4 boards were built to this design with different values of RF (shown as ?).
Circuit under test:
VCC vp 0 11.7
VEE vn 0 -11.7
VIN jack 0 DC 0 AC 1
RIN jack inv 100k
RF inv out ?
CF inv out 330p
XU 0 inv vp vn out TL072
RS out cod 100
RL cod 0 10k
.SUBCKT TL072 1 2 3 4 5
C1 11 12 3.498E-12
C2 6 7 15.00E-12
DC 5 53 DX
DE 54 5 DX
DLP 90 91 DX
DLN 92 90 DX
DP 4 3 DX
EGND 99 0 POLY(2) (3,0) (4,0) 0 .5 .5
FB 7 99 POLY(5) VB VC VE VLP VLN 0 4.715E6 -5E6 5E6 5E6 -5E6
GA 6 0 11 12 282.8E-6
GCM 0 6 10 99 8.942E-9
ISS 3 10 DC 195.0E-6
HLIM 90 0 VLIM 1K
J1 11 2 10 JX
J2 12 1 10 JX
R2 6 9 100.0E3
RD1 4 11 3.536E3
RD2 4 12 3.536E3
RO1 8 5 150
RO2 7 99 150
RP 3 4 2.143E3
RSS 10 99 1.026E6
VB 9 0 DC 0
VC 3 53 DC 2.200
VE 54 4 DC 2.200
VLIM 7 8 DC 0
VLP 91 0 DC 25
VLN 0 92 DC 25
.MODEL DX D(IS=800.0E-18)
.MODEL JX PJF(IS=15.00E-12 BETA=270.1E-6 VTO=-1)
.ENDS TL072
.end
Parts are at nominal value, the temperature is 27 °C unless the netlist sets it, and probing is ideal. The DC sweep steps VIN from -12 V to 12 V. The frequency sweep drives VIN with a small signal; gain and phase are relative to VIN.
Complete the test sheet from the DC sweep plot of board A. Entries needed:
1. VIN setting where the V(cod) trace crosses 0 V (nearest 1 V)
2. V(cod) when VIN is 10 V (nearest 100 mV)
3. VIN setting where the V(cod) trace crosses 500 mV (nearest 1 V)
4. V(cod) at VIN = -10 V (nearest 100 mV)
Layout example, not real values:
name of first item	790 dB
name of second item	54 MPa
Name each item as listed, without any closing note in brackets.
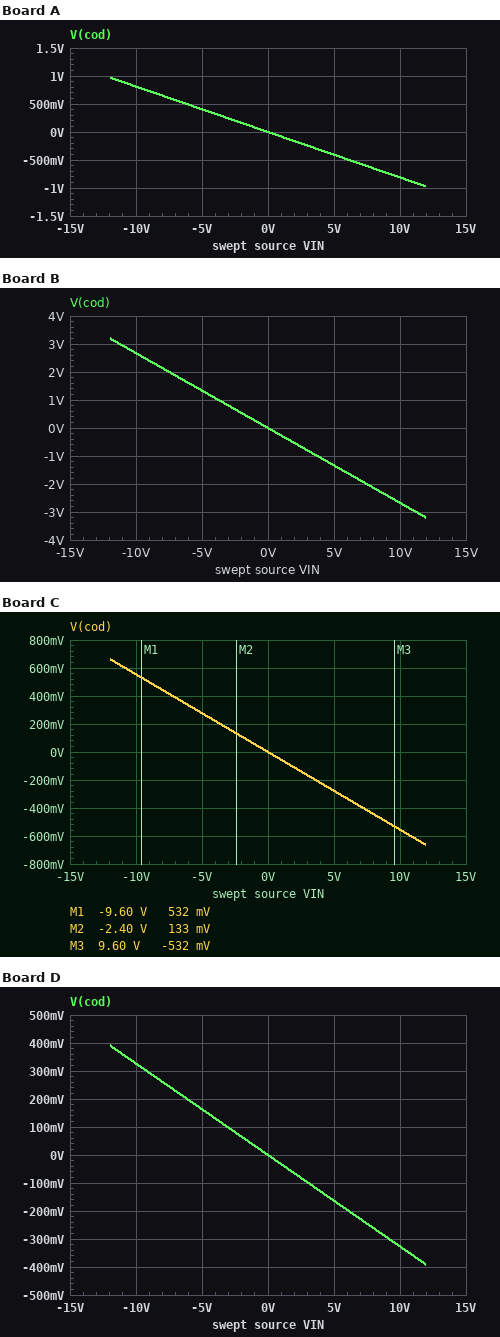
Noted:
VIN setting where the V(cod) trace crosses 0 V	0 V
V(cod) when VIN is 10 V	-800 mV
VIN setting where the V(cod) trace crosses 500 mV	-6 V
V(cod) at VIN = -10 V	800 mV
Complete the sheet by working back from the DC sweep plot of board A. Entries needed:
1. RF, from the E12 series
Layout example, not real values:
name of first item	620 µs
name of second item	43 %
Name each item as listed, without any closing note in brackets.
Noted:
RF, from the E12 series	8.2 kΩ
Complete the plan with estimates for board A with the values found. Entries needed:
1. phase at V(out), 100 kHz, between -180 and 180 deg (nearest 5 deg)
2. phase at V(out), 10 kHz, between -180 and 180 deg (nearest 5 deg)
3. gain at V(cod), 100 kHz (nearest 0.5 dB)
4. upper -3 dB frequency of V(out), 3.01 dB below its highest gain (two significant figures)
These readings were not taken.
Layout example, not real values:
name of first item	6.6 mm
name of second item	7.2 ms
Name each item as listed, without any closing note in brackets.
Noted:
phase at V(out), 100 kHz, between -180 and 180 deg	120 deg
phase at V(out), 10 kHz, between -180 and 180 deg	170 deg
gain at V(cod), 100 kHz	-27.5 dB
upper -3 dB frequency of V(out), 3.01 dB below its highest gain	59 kHz
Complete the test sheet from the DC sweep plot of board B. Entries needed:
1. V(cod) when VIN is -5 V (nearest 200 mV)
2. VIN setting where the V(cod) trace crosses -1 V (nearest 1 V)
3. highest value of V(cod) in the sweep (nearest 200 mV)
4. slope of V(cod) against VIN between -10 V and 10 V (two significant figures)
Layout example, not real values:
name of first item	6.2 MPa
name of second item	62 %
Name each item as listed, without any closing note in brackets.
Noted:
V(cod) when VIN is -5 V	1.4 V
VIN setting where the V(cod) trace crosses -1 V	4 V
highest value of V(cod) in the sweep	3.2 V
slope of V(cod) against VIN between -10 V and 10 V	-0.27 V/V
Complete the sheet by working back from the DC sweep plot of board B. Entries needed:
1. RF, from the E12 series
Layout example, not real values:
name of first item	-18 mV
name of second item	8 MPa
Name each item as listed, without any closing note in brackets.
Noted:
RF, from the E12 series	27 kΩ
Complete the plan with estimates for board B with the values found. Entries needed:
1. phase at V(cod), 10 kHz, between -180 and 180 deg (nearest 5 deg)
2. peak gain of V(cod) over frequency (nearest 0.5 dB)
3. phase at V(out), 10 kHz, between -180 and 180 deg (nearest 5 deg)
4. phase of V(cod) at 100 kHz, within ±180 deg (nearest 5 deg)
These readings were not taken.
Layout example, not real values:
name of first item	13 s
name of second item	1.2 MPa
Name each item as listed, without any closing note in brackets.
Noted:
phase at V(cod), 10 kHz, between -180 and 180 deg	150 deg
peak gain of V(cod) over frequency	-11.5 dB
phase at V(out), 10 kHz, between -180 and 180 deg	150 deg
phase of V(cod) at 100 kHz, within ±180 deg	100 deg
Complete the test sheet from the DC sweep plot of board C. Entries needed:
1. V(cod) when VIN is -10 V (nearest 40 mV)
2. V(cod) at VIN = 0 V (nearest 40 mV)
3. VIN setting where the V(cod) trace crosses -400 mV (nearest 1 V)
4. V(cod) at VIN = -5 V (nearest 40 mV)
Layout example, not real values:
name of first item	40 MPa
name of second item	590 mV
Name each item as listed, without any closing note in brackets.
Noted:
V(cod) when VIN is -10 V	560 mV
V(cod) at VIN = 0 V	0 V
VIN setting where the V(cod) trace crosses -400 mV	7 V
V(cod) at VIN = -5 V	280 mV
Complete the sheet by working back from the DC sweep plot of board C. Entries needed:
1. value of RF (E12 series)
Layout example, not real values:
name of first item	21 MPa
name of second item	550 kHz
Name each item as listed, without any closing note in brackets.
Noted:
value of RF	5.6 kΩ
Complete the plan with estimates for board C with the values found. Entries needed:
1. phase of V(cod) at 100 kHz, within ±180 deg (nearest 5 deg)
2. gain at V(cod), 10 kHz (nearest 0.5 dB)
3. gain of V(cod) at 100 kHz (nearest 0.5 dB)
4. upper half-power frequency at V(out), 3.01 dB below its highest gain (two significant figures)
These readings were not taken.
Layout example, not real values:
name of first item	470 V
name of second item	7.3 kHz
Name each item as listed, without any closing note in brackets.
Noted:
phase of V(cod) at 100 kHz, within ±180 deg	130 deg
gain at V(cod), 10 kHz	-25.0 dB
gain of V(cod) at 100 kHz	-29.0 dB
upper half-power frequency at V(out), 3.01 dB below its highest gain	86 kHz
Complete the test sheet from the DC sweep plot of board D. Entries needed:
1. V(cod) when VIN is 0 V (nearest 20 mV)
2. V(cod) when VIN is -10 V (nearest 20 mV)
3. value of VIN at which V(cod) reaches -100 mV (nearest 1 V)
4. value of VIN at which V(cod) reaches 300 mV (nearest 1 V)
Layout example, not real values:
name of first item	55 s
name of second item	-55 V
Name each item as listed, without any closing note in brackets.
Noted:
V(cod) when VIN is 0 V	0 V
V(cod) when VIN is -10 V	320 mV
value of VIN at which V(cod) reaches -100 mV	3 V
value of VIN at which V(cod) reaches 300 mV	-9 V
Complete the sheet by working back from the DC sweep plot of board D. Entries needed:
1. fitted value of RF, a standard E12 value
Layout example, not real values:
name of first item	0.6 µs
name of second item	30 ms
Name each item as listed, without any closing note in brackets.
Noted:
fitted value of RF, a standard E12 value	3.3 kΩ
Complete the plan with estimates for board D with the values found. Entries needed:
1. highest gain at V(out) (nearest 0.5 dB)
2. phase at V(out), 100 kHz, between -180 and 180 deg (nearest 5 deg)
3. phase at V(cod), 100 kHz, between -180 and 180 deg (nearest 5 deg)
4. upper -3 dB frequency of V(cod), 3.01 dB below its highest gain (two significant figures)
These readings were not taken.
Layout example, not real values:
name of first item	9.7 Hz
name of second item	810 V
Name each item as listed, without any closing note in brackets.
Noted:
highest gain at V(out)	-29.5 dB
phase at V(out), 100 kHz, between -180 and 180 deg	145 deg
phase at V(cod), 100 kHz, between -180 and 180 deg	145 deg
upper -3 dB frequency of V(cod), 3.01 dB below its highest gain	150 kHz
